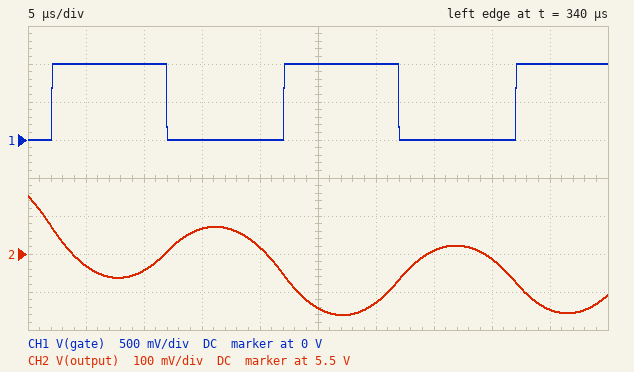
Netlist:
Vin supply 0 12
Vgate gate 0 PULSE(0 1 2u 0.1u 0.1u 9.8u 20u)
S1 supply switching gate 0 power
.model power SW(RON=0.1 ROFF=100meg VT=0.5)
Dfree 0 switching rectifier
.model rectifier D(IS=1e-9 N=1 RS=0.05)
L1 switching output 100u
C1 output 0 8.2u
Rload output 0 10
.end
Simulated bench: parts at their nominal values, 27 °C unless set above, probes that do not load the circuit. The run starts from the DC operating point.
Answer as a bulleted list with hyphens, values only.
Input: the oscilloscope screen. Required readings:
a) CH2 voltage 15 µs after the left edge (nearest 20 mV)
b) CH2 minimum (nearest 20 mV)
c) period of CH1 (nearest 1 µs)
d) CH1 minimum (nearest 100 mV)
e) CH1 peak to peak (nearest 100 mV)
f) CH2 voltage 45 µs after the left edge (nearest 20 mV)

- 5.56 V
- 5.34 V
- 20 µs
- 0 V
- 1.0 V
- 5.36 V
